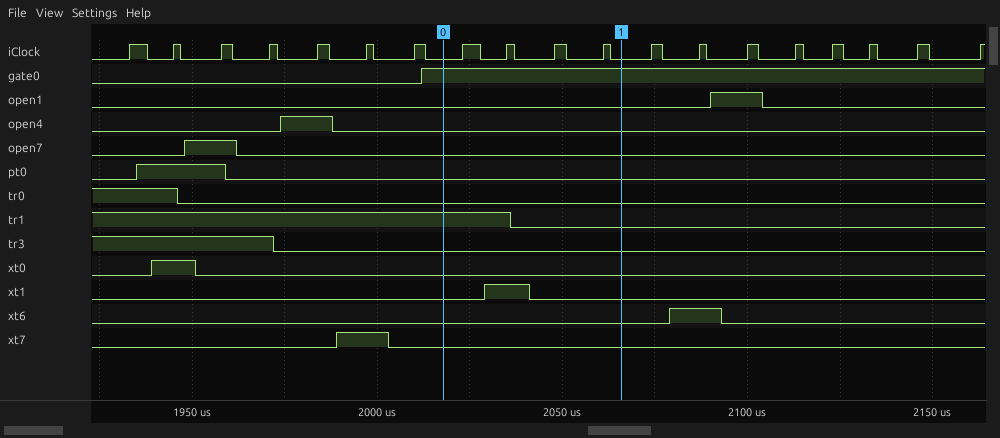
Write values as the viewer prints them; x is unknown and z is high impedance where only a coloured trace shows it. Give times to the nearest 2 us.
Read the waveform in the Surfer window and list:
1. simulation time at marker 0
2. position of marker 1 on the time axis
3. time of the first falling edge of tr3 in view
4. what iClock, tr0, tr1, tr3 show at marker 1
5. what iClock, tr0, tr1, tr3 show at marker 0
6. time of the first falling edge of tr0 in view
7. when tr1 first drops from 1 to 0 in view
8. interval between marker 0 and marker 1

2018 us
2066 us
1972 us
iClock=0, tr0=0, tr1=0, tr3=0
iClock=0, tr0=0, tr1=1, tr3=0
1946 us
2036 us
48 us
